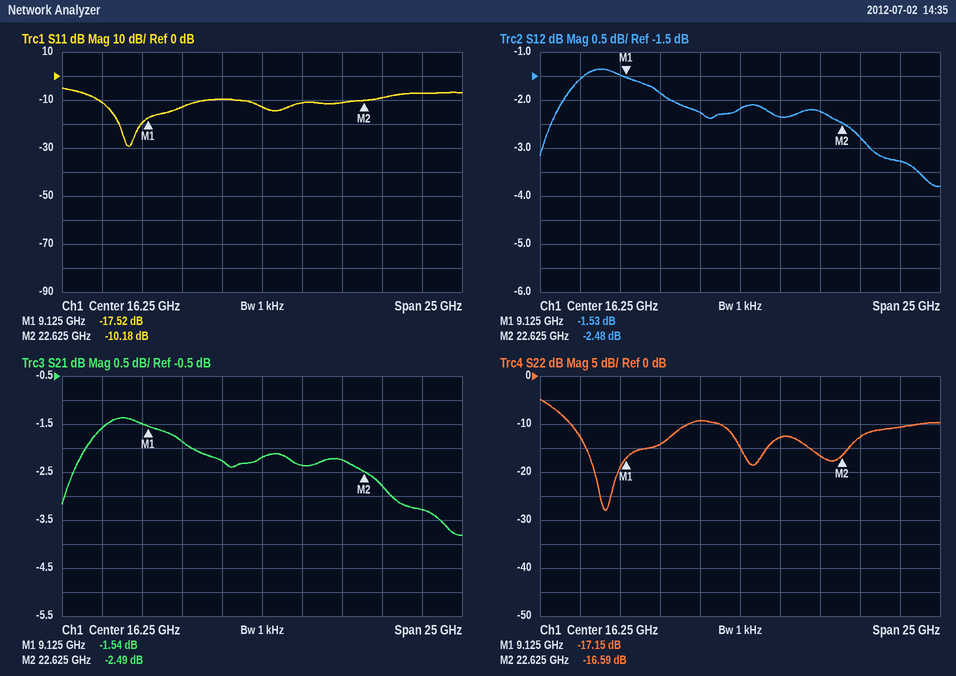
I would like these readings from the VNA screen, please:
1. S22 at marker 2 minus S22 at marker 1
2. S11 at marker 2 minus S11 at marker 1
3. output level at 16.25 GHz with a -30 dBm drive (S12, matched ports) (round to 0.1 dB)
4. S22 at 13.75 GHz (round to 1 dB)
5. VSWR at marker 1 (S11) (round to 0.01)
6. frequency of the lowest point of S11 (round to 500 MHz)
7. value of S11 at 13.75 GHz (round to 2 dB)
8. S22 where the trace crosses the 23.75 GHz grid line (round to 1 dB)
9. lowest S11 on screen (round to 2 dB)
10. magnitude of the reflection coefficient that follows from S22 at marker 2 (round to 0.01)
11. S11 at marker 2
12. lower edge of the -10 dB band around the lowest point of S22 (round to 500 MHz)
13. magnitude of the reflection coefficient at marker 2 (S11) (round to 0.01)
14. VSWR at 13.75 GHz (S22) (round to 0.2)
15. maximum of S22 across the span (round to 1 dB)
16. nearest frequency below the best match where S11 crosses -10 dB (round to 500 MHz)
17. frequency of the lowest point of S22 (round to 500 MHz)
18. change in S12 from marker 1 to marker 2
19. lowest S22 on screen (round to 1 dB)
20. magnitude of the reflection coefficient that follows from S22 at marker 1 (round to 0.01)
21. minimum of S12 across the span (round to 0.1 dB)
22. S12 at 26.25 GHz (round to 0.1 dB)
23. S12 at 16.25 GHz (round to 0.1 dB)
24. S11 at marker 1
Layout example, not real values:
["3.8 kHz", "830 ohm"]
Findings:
["0.56 dB", "7.34 dB", "-32.2 dBm", "-9 dB", "1.31", "8.0 GHz", "-10 dB", "-13 dB", "-30 dB", "0.15", "-10.18 dB", "5.5 GHz", "0.31", "2.0", "-5 dB", "6.0 GHz", "8.0 GHz", "-0.95 dB", "-28 dB", "0.14", "-3.8 dB", "-3.3 dB", "-2.2 dB", "-17.52 dB"]
